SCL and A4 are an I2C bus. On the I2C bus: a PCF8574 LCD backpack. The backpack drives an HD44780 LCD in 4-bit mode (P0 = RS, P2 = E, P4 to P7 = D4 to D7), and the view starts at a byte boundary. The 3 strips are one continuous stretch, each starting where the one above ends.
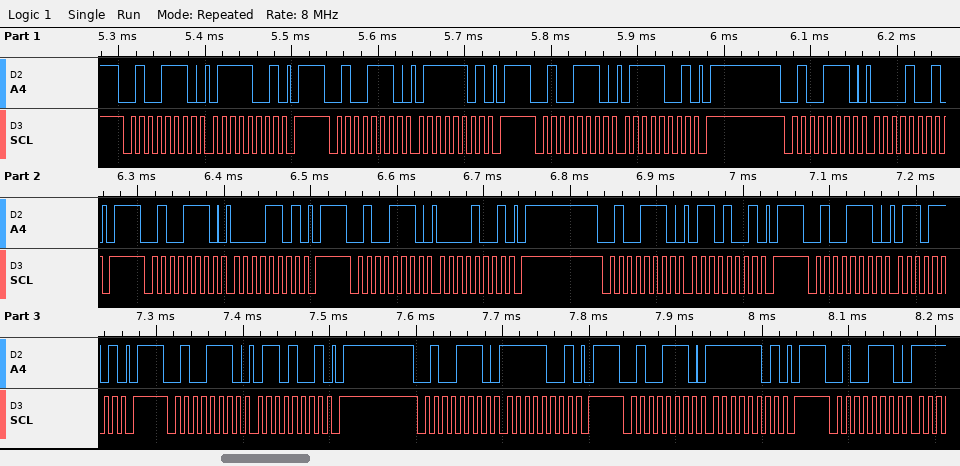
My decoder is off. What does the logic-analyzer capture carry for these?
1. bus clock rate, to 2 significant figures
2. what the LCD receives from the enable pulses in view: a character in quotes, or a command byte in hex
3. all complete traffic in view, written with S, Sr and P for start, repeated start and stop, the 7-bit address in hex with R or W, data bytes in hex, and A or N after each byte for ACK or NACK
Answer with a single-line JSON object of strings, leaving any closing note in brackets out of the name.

{"bus clock rate, to 2 significant figures": "100 kHz", "what the LCD receives from the enable pulses in view: a character in quotes, or a command byte in hex": "'p'", "all complete traffic in view, written with S, Sr and P for start, repeated start and stop, the 7-bit address in hex with R or W, data bytes in hex, and A or N after each byte for ACK or NACK": "S 27W A 79 A P S 27W A 7D A P S 27W A 79 A P S 27W A 09 A P S 27W A 0D A P S 27W A 09 A P S 27W A 69 A P S 27W A 6D A P S 27W A 69 A P S 27W A F9 A P S 27W A FD A P S 27W A"}
